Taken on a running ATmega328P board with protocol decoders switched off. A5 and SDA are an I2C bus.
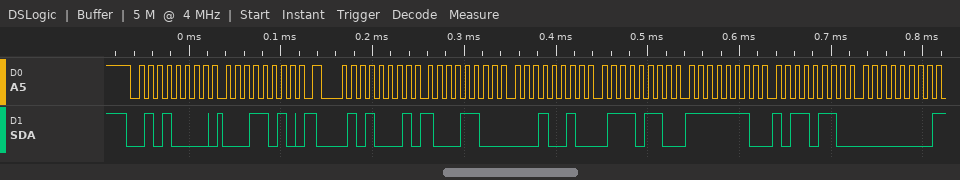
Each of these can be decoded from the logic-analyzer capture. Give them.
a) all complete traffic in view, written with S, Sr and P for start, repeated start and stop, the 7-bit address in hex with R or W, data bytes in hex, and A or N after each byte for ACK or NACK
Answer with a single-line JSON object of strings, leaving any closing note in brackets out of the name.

{"all complete traffic in view, written with S, Sr and P for start, repeated start and stop, the 7-bit address in hex with R or W, data bytes in hex, and A or N after each byte for ACK or NACK": "S 28W A 1A A Sr 28R A 8C A 12 A 76 A FE A B6 A 00 N"}
